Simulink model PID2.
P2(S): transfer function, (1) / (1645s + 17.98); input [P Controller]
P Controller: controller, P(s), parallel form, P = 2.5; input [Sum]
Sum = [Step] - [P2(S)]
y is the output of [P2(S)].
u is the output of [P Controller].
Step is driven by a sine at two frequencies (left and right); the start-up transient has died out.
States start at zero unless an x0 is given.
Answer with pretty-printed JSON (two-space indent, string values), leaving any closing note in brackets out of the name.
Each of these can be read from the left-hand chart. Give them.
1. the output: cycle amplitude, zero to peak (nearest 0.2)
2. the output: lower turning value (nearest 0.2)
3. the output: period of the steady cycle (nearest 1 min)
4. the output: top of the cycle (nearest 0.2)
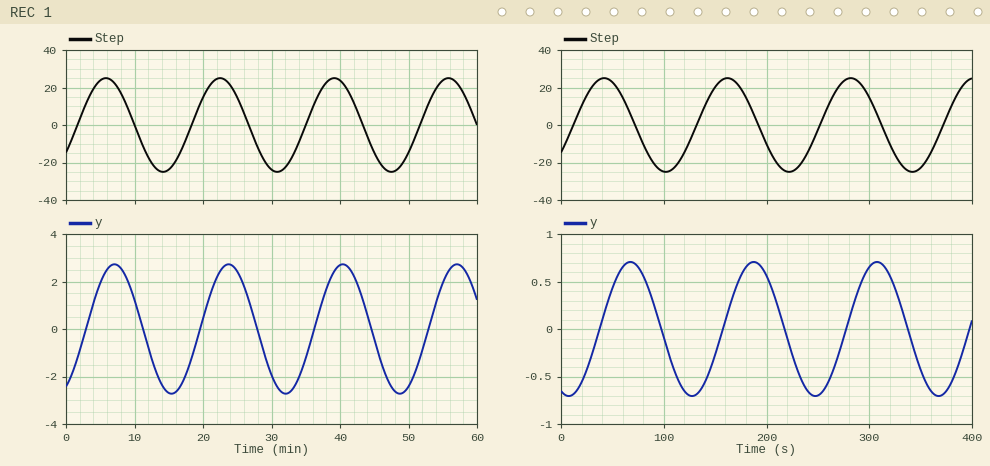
{
  "the output: cycle amplitude, zero to peak": "2.8",
  "the output: lower turning value": "-2.8",
  "the output: period of the steady cycle": "17 min",
  "the output: top of the cycle": "2.8"
}
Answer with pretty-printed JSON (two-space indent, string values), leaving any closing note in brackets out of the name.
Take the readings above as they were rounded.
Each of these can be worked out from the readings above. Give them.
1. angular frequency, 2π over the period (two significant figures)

{
  "angular frequency, 2π over the period": "0.37 rad/min"
}
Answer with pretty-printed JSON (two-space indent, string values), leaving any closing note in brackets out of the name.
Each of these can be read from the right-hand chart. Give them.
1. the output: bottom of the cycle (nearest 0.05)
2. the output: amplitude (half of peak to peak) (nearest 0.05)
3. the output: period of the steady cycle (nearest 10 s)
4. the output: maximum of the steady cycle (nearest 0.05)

{
  "the output: bottom of the cycle": "-0.70",
  "the output: amplitude (half of peak to peak)": "0.70",
  "the output: period of the steady cycle": "120 s",
  "the output: maximum of the steady cycle": "0.70"
}
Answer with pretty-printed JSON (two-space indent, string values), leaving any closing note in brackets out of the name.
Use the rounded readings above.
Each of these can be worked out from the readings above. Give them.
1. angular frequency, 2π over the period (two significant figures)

{
  "angular frequency, 2π over the period": "0.052 rad/s"
}
